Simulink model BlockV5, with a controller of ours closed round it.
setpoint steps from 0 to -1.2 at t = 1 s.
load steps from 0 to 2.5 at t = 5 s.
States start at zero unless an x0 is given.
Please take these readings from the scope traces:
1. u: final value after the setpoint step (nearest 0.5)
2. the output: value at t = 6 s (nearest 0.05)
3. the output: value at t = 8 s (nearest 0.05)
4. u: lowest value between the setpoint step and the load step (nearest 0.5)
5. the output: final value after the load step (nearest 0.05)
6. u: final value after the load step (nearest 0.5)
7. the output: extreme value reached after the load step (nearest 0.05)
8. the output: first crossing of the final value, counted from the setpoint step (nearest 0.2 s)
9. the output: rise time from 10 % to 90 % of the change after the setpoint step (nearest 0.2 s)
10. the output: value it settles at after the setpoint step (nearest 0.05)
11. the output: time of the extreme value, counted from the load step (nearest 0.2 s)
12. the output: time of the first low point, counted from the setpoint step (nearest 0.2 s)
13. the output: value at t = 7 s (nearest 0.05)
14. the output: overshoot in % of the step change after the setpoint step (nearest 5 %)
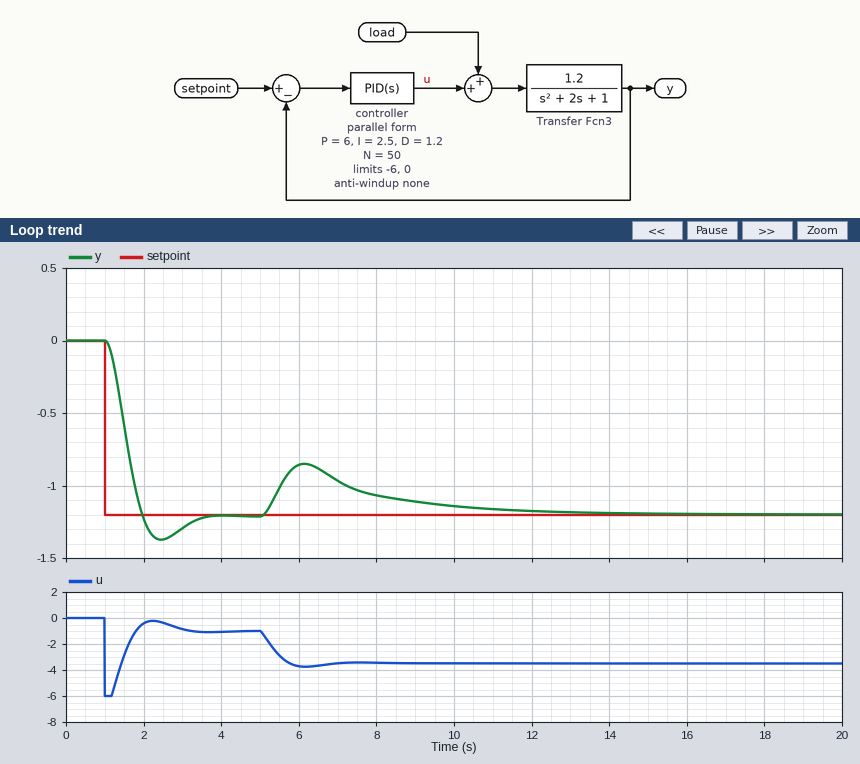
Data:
-1.0
-0.85
-1.05
-6.0
-1.20
-3.5
-0.85
1.0 s
0.6 s
-1.20
1.2 s
1.4 s
-0.95
15 %
